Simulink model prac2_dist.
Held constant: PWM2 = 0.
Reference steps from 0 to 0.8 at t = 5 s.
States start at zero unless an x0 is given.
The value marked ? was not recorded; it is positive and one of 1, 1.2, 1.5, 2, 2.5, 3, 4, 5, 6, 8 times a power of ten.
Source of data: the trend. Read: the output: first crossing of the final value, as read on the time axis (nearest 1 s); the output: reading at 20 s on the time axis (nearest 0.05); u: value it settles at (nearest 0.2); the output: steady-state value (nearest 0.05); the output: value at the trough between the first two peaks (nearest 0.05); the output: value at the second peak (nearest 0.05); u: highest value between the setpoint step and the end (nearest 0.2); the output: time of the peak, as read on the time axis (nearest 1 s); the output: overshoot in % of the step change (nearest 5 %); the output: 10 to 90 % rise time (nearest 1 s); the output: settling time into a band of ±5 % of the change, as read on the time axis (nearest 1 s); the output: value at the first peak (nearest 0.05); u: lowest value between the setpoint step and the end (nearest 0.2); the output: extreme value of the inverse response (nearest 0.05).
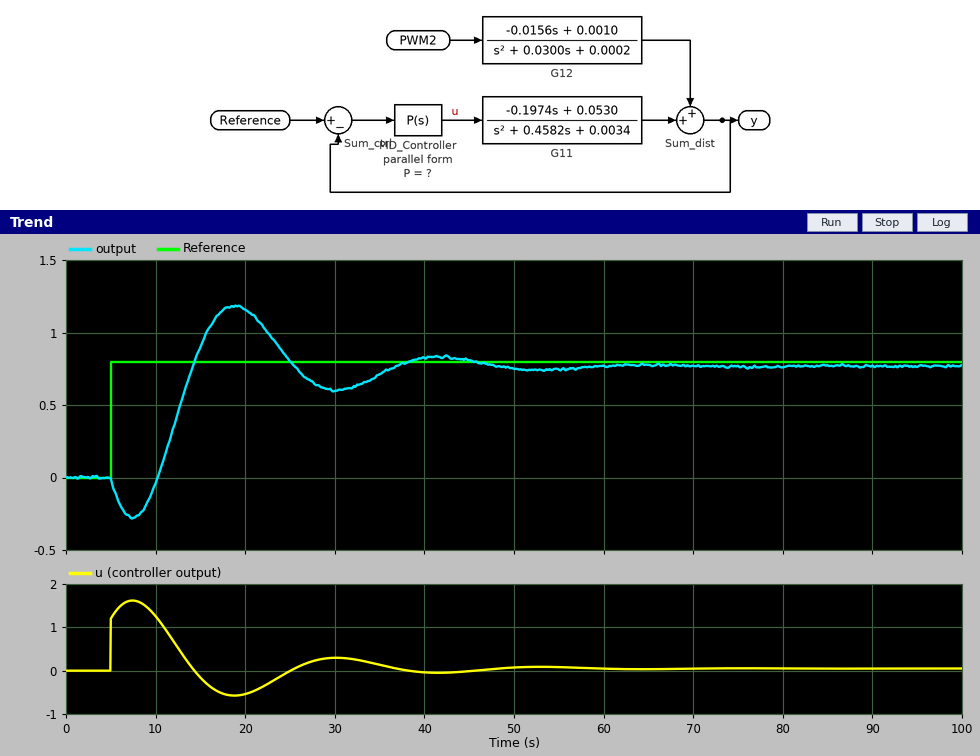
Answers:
14 s
1.15
0.0
0.75
0.60
0.85
1.6
19 s
55 %
3 s
45 s
1.20
-0.6
-0.30
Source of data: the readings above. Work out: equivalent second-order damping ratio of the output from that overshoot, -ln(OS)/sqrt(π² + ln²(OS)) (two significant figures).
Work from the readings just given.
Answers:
0.19
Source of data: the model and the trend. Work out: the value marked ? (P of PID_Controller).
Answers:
1.5
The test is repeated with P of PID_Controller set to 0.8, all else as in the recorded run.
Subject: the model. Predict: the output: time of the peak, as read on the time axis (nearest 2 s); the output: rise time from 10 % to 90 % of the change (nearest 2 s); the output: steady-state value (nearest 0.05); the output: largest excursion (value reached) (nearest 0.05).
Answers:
28 s
8 s
0.75
0.80
